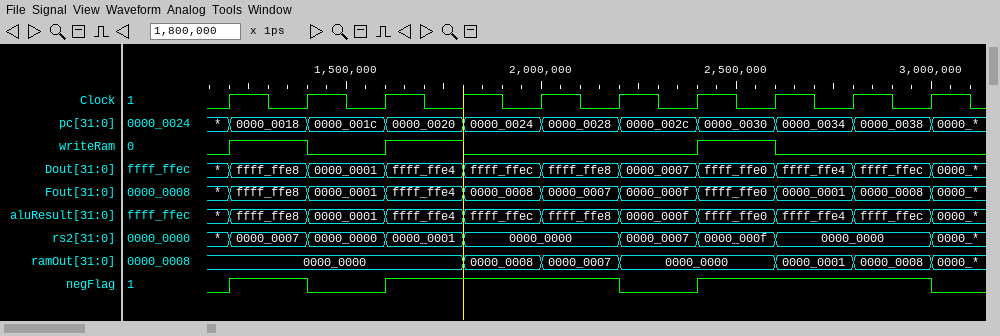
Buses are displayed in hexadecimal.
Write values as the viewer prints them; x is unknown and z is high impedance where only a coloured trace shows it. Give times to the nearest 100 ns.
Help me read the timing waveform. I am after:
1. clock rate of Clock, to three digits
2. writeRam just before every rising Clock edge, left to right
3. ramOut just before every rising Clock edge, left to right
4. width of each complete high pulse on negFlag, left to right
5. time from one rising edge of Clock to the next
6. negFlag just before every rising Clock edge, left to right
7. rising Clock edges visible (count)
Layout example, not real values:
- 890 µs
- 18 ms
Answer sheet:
- 5.00 MHz
- 0 1 0 1 0 0 0 1 0 0
- 0000_0000, 0000_0000, 0000_0000, 0000_0000, 0000_0008, 0000_0007, 0000_0000, 0000_0000, 0000_0001, 0000_0008
- 200 ns, 600 ns, 600 ns
- 200 ns
- 0 1 0 1 1 1 0 1 1 1
- 10
